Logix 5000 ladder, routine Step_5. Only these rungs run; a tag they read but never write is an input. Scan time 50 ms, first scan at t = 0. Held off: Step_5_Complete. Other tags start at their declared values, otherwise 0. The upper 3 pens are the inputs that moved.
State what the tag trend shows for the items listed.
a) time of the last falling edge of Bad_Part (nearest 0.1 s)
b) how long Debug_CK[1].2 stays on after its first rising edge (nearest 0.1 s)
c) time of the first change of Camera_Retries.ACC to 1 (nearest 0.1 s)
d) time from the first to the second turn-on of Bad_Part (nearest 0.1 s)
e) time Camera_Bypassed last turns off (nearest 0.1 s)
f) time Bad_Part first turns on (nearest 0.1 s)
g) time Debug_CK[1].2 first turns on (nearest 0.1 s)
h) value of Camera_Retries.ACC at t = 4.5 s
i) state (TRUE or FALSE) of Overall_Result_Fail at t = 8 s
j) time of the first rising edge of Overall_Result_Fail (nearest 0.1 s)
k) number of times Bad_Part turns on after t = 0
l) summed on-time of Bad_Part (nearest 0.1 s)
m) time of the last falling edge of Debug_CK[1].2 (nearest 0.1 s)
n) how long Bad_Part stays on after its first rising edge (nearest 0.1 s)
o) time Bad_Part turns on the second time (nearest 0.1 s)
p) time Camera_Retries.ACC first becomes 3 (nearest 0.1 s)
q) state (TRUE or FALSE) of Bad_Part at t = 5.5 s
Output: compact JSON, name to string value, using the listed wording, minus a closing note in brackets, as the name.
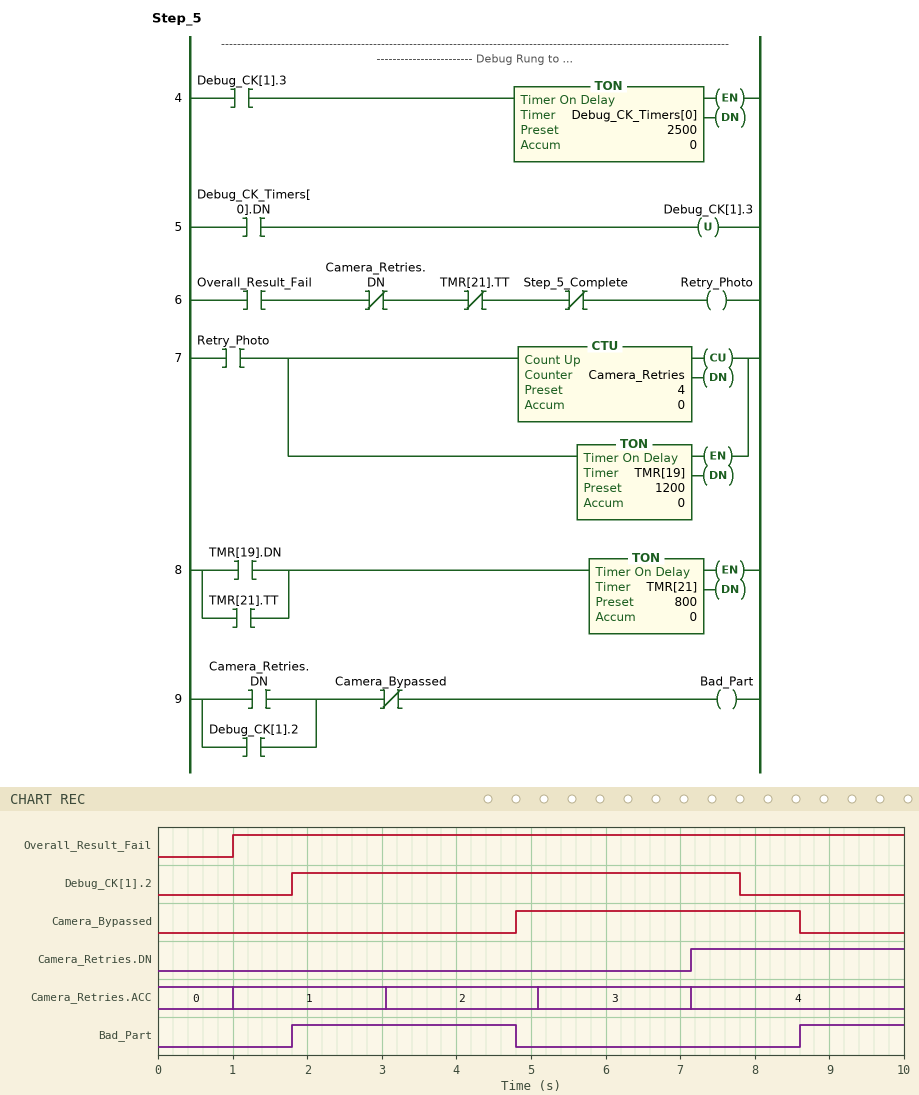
{"time of the last falling edge of Bad_Part": "4.8 s", "how long Debug_CK[1].2 stays on after its first rising edge": "6.0 s", "time of the first change of Camera_Retries.ACC to 1": "1.0 s", "time from the first to the second turn-on of Bad_Part": "6.8 s", "time Camera_Bypassed last turns off": "8.6 s", "time Bad_Part first turns on": "1.8 s", "time Debug_CK[1].2 first turns on": "1.8 s", "value of Camera_Retries.ACC at t = 4.5 s": "2", "state (TRUE or FALSE) of Overall_Result_Fail at t = 8 s": "TRUE", "time of the first rising edge of Overall_Result_Fail": "1.0 s", "number of times Bad_Part turns on after t = 0": "2", "summed on-time of Bad_Part": "4.4 s", "time of the last falling edge of Debug_CK[1].2": "7.8 s", "how long Bad_Part stays on after its first rising edge": "3.0 s", "time Bad_Part turns on the second time": "8.6 s", "time Camera_Retries.ACC first becomes 3": "5.1 s", "state (TRUE or FALSE) of Bad_Part at t = 5.5 s": "FALSE"}
